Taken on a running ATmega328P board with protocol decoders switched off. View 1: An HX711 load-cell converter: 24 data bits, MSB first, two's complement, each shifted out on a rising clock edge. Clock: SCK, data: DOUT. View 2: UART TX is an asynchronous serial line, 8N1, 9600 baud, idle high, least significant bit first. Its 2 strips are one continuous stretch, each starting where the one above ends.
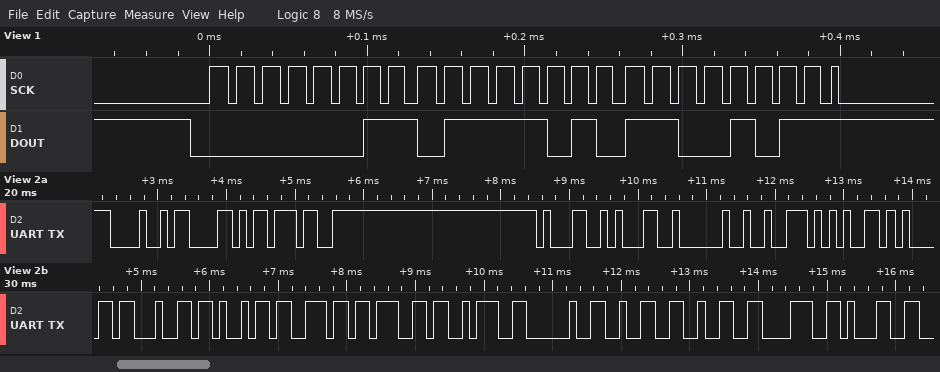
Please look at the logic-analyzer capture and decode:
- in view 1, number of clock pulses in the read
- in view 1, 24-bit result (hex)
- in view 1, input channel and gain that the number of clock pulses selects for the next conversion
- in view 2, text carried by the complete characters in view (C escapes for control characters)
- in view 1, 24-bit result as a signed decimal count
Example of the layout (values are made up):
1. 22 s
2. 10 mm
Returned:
1. 25
2. 0x037ACB
3. channel A, gain 128
4. "HX711 reading: 2281"
5. 228043
